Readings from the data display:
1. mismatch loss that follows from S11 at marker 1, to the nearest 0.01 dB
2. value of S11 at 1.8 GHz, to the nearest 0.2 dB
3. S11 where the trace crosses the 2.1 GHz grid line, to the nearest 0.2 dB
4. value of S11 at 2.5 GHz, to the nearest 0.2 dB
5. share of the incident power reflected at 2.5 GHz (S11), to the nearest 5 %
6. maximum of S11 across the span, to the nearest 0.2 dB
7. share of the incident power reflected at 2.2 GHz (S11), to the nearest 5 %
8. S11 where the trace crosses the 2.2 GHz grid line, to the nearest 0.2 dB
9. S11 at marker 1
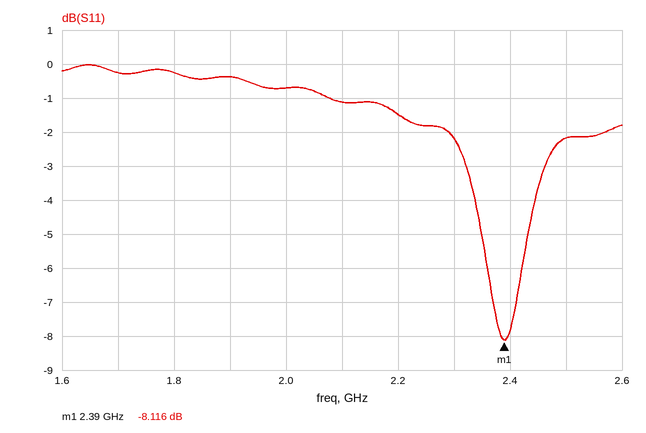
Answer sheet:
0.73 dB
-0.2 dB
-1.2 dB
-2.2 dB
60 %
0.0 dB
70 %
-1.4 dB
-8.116 dB
